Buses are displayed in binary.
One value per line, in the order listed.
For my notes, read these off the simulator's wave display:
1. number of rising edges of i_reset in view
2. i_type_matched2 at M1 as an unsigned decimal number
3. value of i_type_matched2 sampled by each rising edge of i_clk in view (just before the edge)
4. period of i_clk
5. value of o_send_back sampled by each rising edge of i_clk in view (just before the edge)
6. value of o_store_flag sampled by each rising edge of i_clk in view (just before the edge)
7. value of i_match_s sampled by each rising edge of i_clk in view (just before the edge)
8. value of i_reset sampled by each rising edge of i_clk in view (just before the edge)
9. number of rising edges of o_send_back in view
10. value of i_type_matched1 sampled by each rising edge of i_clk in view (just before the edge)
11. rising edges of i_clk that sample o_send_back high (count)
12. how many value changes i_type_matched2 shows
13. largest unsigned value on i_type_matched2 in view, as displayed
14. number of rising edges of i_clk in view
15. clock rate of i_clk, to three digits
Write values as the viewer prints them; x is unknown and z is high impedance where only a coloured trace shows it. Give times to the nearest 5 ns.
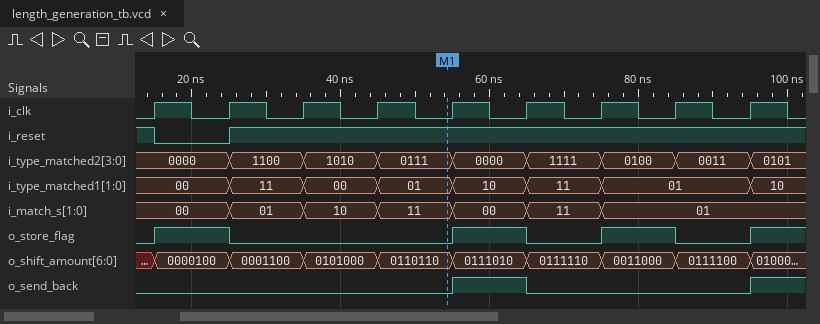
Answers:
1
7
0000, 0000, 1100, 1010, 0111, 0000, 1111, 0100, 0011
10 ns
0 0 0 0 0 1 0 0 0
0 1 0 0 0 1 0 1 0
00, 00, 01, 10, 11, 00, 11, 01, 01
1 0 1 1 1 1 1 1 1
2
00, 00, 11, 00, 01, 10, 11, 01, 01
1
8
1111
9
100 MHz
